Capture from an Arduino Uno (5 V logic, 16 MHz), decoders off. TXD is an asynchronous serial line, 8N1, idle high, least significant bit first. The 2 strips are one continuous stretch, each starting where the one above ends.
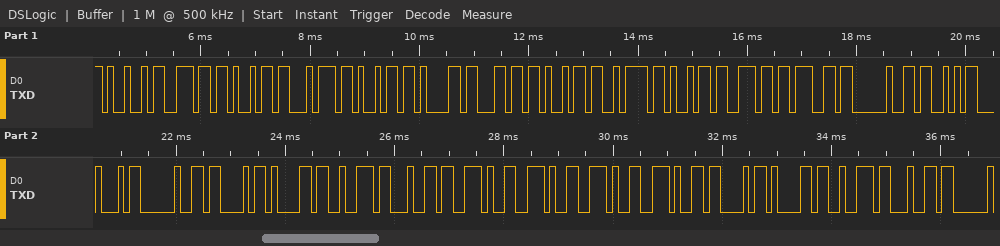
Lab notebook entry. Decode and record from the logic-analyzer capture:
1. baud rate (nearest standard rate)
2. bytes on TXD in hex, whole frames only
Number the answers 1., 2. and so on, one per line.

1. 9600 baud
2. 49 6E 69 74 69 61 6C 69 7A 69 6E 67 20 53 44 20 43 61 72 64 2E 2E 2E 2E 43 61 72 64
